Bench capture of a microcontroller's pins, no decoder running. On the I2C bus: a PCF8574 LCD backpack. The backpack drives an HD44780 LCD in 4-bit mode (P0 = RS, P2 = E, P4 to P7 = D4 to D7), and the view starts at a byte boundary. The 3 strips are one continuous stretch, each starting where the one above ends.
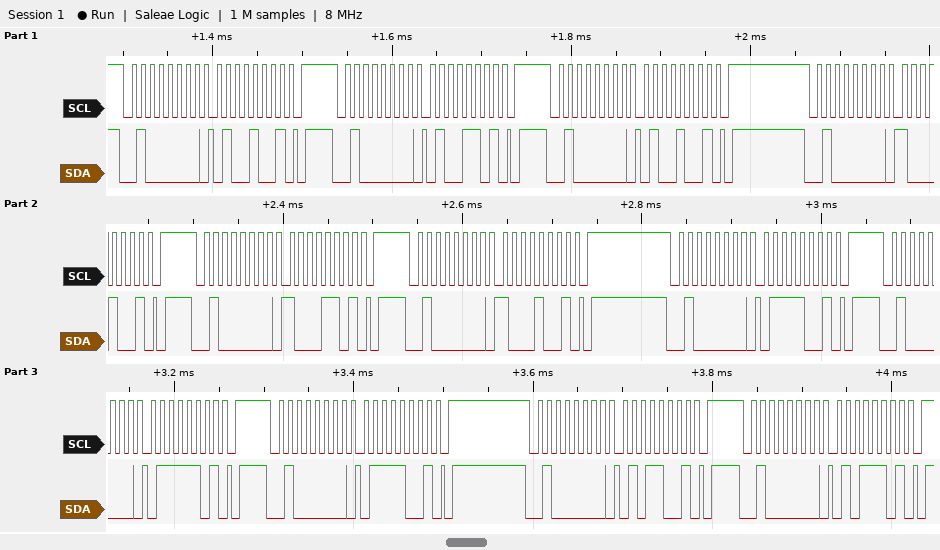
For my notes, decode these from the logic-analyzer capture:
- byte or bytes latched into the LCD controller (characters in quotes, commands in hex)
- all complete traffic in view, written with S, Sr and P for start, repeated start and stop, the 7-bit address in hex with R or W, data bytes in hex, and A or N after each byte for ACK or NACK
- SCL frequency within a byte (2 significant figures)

'H'
S 20W A 49 A P S 20W A 4D A P S 20W A 49 A P S 20W A 89 A P S 20W A 8D A P S 20W A 89 A P S 20W A 79 A P S 20W A 7D A P S 20W A 79 A P S 20W A 59 A P S 20W A 5D A P
100 kHz
